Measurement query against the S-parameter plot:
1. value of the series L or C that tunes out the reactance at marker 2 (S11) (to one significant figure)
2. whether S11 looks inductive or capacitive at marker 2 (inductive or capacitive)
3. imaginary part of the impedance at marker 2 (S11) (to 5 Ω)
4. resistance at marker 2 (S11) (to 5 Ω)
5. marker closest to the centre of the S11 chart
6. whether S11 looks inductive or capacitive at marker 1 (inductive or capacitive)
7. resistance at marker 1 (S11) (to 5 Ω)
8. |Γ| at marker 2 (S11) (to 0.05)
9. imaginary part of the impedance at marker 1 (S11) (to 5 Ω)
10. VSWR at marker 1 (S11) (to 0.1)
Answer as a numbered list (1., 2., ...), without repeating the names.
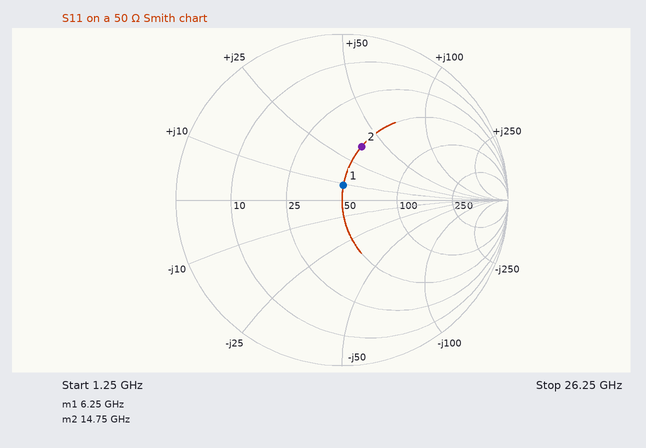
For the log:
1. 300 fF
2. inductive
3. +35 Ω
4. 50 Ω
5. marker 1
6. inductive
7. 50 Ω
8. 0.35
9. +10 Ω
10. 1.2
